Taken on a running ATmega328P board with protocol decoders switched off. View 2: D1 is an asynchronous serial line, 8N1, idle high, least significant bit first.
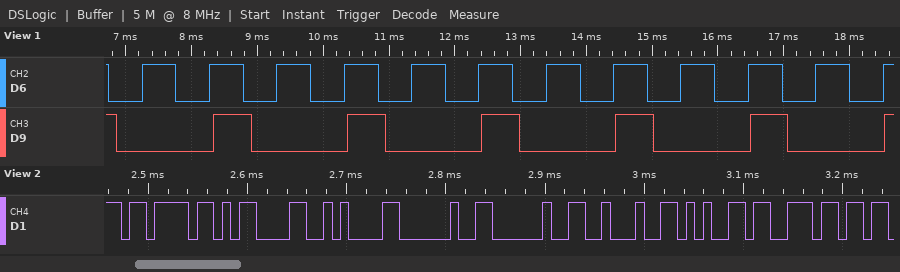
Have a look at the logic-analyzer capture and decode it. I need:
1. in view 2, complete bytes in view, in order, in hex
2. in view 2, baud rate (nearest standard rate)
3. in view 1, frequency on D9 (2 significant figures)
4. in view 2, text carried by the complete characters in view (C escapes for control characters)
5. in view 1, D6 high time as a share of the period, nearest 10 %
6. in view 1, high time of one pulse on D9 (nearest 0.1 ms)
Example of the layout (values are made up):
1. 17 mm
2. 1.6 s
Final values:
1. 7B 0D 0A 20 20 22 65 6E
2. 115200 baud
3. 490 Hz
4. "{\r\n  \"en"
5. 50 %
6. 0.6 ms
